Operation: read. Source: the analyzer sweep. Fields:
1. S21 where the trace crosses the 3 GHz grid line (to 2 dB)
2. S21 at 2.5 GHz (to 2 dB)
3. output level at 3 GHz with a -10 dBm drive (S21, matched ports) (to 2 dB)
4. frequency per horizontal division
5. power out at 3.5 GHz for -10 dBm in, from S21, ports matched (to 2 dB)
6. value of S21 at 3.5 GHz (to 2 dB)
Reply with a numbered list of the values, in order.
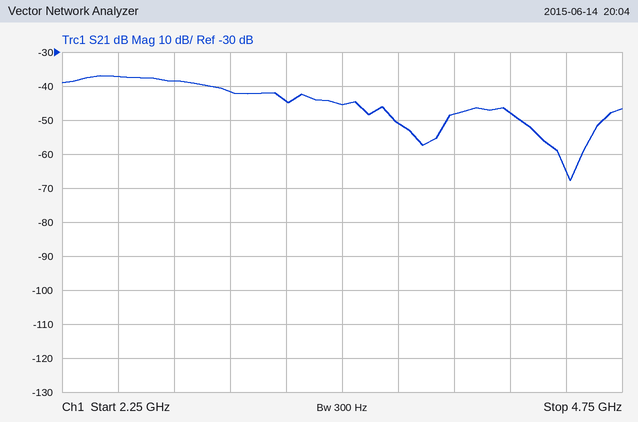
1. -42 dB
2. -38 dB
3. -52 dBm
4. 250 MHz
5. -56 dBm
6. -46 dB
